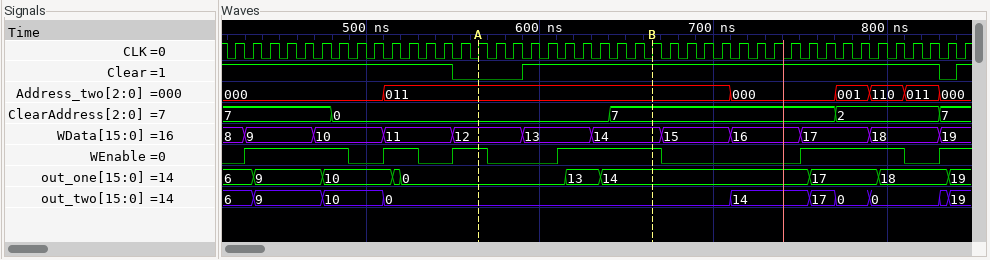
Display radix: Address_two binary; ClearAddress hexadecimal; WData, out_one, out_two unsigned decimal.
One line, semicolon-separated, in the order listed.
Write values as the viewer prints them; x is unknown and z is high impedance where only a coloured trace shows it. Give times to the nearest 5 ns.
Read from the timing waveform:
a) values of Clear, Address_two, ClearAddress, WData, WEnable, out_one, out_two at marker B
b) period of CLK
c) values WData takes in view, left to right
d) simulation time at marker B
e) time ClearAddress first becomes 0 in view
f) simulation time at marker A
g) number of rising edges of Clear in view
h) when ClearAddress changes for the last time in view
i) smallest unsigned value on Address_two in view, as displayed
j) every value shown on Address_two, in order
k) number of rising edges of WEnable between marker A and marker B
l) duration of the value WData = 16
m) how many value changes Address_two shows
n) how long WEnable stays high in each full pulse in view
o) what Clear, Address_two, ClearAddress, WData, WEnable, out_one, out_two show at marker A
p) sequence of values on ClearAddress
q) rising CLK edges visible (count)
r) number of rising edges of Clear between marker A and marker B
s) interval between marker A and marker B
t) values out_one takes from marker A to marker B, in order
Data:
Clear=1, Address_two=011, ClearAddress=7, WData=14, WEnable=1, out_one=14, out_two=0; 10 ns; 8, 9, 10, 11, 12, 13, 14, 15, 16, 17, 18, 19; 665 ns; 480 ns; 565 ns; 2; 830 ns; 000; 000, 011, 000, 001, 110, 011, 000; 1; 40 ns; 6; 60 ns, 20 ns, 20 ns, 60 ns, 60 ns; Clear=0, Address_two=011, ClearAddress=0, WData=12, WEnable=1, out_one=0, out_two=0; 7, 0, 7, 2, 7; 43; 1; 100 ns; 0, 13, 14
